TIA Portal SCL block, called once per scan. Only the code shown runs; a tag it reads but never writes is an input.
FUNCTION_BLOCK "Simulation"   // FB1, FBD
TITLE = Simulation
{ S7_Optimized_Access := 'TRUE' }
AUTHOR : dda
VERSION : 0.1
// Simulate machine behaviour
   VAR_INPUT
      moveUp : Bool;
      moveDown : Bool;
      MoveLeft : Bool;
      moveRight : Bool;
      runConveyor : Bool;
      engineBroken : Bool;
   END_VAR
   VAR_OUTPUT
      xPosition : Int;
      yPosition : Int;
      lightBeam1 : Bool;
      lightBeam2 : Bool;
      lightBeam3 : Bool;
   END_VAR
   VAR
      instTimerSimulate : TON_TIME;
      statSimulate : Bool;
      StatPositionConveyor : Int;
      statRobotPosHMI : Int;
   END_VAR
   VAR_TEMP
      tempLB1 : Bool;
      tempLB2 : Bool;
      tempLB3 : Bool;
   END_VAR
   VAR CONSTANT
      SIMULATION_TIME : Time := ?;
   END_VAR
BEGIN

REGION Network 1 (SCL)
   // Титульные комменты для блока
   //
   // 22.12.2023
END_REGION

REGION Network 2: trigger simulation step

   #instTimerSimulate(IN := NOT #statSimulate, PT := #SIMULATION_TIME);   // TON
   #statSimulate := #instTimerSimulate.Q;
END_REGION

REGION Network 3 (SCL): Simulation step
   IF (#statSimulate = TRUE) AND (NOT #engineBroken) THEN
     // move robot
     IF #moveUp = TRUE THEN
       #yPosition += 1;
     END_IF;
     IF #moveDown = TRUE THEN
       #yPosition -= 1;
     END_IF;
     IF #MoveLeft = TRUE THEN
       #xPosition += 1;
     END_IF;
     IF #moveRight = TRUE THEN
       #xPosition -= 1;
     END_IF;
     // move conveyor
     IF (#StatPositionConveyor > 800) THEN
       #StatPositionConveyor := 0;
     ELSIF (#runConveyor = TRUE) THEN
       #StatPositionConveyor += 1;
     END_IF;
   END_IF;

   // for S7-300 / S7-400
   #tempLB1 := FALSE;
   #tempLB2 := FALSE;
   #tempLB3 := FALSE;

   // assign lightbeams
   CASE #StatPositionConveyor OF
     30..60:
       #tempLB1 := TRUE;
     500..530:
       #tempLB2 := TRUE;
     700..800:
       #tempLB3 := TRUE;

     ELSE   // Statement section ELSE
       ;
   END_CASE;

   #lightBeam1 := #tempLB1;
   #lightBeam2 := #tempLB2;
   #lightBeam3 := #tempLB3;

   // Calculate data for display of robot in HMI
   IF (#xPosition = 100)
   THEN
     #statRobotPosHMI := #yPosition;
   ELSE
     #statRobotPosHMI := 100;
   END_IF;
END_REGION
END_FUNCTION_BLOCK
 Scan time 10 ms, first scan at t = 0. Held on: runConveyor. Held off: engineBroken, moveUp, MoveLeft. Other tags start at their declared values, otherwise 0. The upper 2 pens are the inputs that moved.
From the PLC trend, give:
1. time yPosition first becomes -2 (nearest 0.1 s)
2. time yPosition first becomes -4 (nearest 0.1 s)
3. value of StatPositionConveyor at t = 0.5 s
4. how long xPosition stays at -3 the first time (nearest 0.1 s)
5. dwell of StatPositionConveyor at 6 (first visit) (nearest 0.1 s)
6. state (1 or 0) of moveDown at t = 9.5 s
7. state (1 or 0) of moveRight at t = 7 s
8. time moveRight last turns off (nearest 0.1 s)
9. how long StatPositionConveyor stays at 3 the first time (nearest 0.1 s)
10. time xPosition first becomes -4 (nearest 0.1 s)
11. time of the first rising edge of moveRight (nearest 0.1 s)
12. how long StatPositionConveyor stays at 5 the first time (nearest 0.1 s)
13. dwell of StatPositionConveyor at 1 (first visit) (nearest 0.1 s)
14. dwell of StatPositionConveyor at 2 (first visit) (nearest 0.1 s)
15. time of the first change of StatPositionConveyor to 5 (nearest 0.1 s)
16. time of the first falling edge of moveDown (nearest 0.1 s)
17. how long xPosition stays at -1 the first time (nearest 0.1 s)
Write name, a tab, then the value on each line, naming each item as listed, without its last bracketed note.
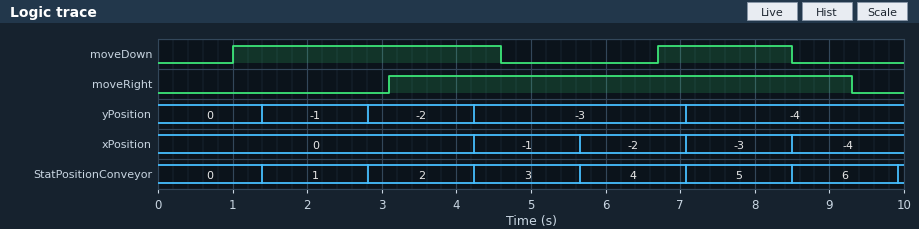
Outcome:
time yPosition first becomes -2	2.8 s
time yPosition first becomes -4	7.1 s
value of StatPositionConveyor at t = 0.5 s	0
how long xPosition stays at -3 the first time	1.4 s
dwell of StatPositionConveyor at 6 (first visit)	1.4 s
state (1 or 0) of moveDown at t = 9.5 s	0
state (1 or 0) of moveRight at t = 7 s	1
time moveRight last turns off	9.3 s
how long StatPositionConveyor stays at 3 the first time	1.4 s
time xPosition first becomes -4	8.5 s
time of the first rising edge of moveRight	3.1 s
how long StatPositionConveyor stays at 5 the first time	1.4 s
dwell of StatPositionConveyor at 1 (first visit)	1.4 s
dwell of StatPositionConveyor at 2 (first visit)	1.4 s
time of the first change of StatPositionConveyor to 5	7.1 s
time of the first falling edge of moveDown	4.6 s
how long xPosition stays at -1 the first time	1.4 s
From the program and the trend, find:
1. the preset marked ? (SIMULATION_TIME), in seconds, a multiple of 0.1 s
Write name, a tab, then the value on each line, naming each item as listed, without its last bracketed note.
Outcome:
the preset marked ? (SIMULATION_TIME), in seconds, a multiple of 0.1 s	1.4 s
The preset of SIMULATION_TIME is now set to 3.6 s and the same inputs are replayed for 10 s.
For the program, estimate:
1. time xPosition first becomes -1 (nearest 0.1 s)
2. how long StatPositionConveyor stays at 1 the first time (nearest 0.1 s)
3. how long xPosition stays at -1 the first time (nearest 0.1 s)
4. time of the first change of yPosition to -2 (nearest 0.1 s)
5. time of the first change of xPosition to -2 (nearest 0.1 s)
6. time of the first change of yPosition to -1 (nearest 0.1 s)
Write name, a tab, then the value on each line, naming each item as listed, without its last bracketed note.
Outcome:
time xPosition first becomes -1	3.6 s
how long StatPositionConveyor stays at 1 the first time	3.6 s
how long xPosition stays at -1 the first time	3.6 s
time of the first change of yPosition to -2	7.2 s
time of the first change of xPosition to -2	7.2 s
time of the first change of yPosition to -1	3.6 s
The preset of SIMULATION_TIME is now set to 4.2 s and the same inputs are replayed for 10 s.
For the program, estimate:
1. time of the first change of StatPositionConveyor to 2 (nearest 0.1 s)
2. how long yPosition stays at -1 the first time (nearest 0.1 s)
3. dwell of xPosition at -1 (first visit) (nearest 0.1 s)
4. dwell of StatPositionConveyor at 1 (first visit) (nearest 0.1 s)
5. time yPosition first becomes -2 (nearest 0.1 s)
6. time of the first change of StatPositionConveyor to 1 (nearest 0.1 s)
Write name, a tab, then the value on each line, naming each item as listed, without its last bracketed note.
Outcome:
time of the first change of StatPositionConveyor to 2	8.4 s
how long yPosition stays at -1 the first time	4.2 s
dwell of xPosition at -1 (first visit)	4.2 s
dwell of StatPositionConveyor at 1 (first visit)	4.2 s
time yPosition first becomes -2	8.4 s
time of the first change of StatPositionConveyor to 1	4.2 s
